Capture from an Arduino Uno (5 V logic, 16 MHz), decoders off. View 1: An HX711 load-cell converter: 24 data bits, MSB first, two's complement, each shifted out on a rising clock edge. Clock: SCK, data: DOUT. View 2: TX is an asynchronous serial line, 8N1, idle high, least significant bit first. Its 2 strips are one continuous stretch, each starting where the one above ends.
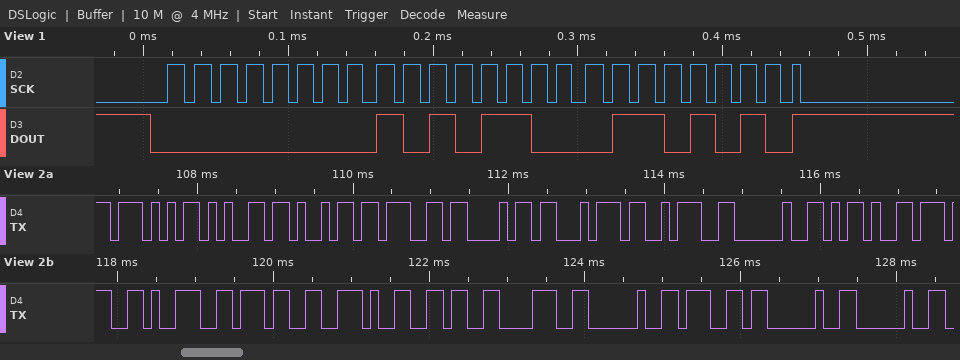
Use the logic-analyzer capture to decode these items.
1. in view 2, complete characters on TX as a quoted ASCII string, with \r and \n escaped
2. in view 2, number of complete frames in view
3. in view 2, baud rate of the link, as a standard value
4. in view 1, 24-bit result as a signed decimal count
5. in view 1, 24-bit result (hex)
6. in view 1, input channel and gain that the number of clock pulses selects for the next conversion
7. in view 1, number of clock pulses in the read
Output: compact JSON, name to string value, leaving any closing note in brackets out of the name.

{"in view 2, complete characters on TX as a quoted ASCII string, with \\r and \\n escaped": "\"Weight: -797.68 g  \"", "in view 2, number of complete frames in view": "19", "in view 2, baud rate of the link, as a standard value": "9600 baud", "in view 1, 24-bit result as a signed decimal count": "44138", "in view 1, 24-bit result": "0x00AC6A", "in view 1, input channel and gain that the number of clock pulses selects for the next conversion": "channel A, gain 128", "in view 1, number of clock pulses in the read": "25"}
